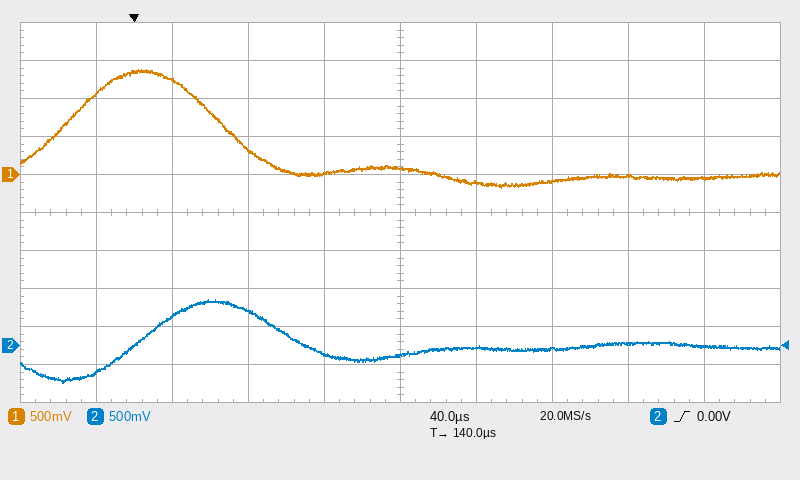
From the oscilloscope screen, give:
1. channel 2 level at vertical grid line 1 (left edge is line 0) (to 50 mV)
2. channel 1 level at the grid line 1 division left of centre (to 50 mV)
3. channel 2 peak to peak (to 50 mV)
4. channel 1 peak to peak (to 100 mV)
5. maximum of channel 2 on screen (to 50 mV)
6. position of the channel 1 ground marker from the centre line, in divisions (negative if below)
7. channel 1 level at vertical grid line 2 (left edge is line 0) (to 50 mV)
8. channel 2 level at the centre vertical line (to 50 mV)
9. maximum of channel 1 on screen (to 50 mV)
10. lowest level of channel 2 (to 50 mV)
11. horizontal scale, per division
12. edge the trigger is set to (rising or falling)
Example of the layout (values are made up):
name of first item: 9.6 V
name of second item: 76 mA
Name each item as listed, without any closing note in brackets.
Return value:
channel 2 level at vertical grid line 1 (left edge is line 0): -350 mV
channel 1 level at the grid line 1 division left of centre: 0 mV
channel 2 peak to peak: 1.10 V
channel 1 peak to peak: 1.60 V
maximum of channel 2 on screen: 600 mV
position of the channel 1 ground marker from the centre line, in divisions: +1.0 div
channel 1 level at vertical grid line 2 (left edge is line 0): 1.25 V
channel 2 level at the centre vertical line: -150 mV
maximum of channel 1 on screen: 1.40 V
lowest level of channel 2: -500 mV
horizontal scale, per division: 40 µs
edge the trigger is set to: rising
